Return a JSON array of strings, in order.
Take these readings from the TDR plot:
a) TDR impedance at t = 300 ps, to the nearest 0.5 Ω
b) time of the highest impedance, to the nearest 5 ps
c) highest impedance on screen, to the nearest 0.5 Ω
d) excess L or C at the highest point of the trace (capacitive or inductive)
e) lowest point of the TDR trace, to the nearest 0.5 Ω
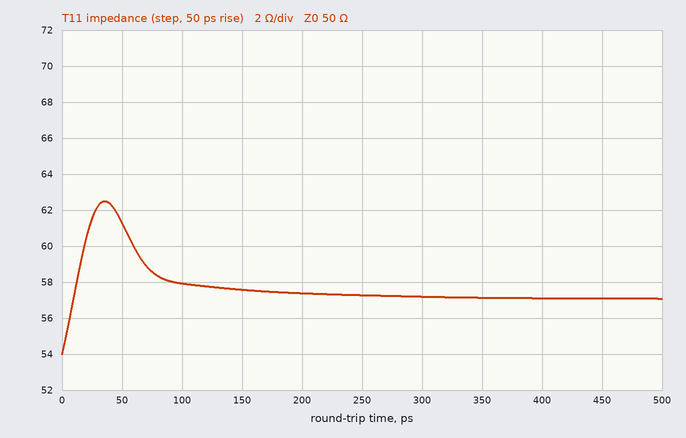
["57.0 Ω", "35 ps", "62.5 Ω", "inductive", "54.0 Ω"]
